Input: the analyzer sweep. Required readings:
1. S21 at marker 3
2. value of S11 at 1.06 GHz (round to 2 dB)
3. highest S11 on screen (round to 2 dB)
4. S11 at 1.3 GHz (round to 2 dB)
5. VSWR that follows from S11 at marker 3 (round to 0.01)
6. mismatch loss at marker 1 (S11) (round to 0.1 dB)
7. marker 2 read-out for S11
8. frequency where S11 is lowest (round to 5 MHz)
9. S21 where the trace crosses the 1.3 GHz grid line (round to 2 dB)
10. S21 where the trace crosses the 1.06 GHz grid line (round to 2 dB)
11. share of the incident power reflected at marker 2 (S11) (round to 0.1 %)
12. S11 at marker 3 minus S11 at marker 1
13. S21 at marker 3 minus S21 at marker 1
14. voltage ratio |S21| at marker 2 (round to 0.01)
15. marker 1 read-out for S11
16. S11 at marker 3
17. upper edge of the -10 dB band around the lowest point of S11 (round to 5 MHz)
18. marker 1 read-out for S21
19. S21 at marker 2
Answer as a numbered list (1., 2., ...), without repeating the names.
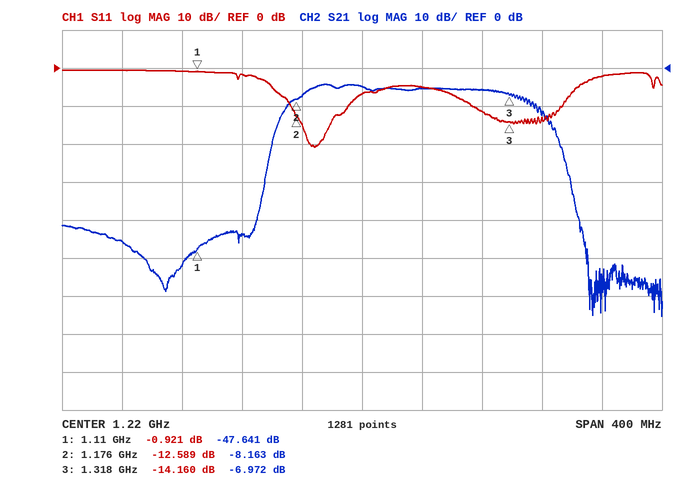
1. -6.972 dB
2. 0 dB
3. 0 dB
4. -12 dB
5. 1.49
6. 7.2 dB
7. -12.589 dB
8. 1.190 GHz
9. -6 dB
10. -46 dB
11. 5.5 %
12. -13.239 dB
13. 40.669 dB
14. 0.39
15. -0.921 dB
16. -14.160 dB
17. 1.210 GHz
18. -47.641 dB
19. -8.163 dB
